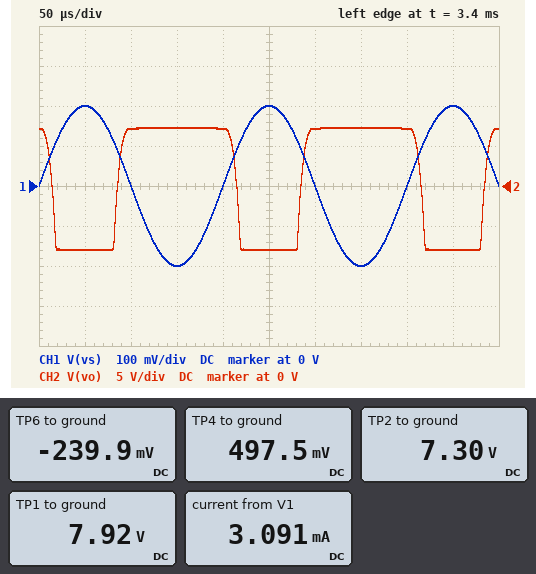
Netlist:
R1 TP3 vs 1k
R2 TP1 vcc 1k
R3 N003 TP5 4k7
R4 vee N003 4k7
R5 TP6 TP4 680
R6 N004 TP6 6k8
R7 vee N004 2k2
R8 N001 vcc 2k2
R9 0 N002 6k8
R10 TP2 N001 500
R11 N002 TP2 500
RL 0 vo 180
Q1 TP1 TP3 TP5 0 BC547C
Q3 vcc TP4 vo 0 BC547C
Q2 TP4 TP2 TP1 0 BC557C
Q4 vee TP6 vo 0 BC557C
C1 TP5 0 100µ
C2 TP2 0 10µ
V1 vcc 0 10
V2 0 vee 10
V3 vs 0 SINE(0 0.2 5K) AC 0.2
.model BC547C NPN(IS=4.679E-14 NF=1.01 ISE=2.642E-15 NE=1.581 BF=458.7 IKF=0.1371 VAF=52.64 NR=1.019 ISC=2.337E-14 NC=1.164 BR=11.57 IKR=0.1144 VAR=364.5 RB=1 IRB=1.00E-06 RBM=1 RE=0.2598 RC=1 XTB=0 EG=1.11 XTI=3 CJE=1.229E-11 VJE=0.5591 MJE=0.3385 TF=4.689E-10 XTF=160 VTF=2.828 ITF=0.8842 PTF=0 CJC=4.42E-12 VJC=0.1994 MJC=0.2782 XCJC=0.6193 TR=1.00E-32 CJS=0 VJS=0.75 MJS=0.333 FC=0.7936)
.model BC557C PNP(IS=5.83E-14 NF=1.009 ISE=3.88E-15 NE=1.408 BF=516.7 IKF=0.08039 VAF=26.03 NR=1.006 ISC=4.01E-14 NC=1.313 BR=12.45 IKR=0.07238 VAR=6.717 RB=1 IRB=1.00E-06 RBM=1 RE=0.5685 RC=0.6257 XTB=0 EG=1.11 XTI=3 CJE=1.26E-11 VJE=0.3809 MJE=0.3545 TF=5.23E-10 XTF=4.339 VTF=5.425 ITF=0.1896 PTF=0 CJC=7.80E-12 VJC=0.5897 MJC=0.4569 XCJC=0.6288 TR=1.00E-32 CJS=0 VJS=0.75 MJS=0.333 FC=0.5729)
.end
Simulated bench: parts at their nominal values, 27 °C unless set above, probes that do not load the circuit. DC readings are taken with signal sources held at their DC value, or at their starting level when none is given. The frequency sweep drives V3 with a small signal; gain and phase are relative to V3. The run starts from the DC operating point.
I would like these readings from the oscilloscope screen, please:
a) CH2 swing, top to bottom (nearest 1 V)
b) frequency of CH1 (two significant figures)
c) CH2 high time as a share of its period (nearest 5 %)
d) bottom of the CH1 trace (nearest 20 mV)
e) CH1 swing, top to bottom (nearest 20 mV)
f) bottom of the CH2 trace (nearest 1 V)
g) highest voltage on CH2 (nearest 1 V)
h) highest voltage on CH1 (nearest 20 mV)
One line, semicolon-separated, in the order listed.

15 V; 5.0 kHz; 65 %; -200 mV; 400 mV; -8 V; 7 V; 200 mV
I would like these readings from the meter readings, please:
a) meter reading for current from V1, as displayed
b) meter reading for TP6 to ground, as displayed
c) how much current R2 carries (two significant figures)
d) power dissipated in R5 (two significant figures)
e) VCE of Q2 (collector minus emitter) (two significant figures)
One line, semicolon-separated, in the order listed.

3.091 mA; -239.9 mV; 2.1 mA; 800 µW; -7.4 V
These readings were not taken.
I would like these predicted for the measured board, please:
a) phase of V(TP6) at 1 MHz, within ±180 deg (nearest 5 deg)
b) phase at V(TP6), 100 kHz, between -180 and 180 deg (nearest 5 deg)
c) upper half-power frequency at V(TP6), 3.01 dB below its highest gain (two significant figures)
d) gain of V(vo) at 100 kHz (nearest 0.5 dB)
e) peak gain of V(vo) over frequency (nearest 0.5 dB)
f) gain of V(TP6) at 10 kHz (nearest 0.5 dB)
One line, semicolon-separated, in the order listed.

95 deg; 165 deg; 370 kHz; 26.0 dB; 26.0 dB; 49.5 dB
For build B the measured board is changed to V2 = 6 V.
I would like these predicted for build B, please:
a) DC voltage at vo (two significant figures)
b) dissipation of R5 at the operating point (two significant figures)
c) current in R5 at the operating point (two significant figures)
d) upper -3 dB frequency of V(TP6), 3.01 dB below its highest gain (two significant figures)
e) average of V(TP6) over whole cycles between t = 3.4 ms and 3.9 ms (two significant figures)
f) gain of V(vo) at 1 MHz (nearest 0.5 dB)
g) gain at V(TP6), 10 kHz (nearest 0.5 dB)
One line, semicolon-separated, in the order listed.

6.7 V; 1.3 mW; 1.4 mA; 1.1 MHz; 3.2 V; 41.5 dB; 43.5 dB
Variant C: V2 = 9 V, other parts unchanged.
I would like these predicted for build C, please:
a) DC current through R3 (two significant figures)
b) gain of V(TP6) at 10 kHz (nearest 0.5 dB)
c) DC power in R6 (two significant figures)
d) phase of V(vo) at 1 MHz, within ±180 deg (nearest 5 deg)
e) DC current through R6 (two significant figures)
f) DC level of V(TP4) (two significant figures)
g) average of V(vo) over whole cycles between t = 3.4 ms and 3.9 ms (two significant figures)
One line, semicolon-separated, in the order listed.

890 µA; 48.0 dB; 9.3 mW; 140 deg; 1.2 mA; 2.3 V; 2.2 V
